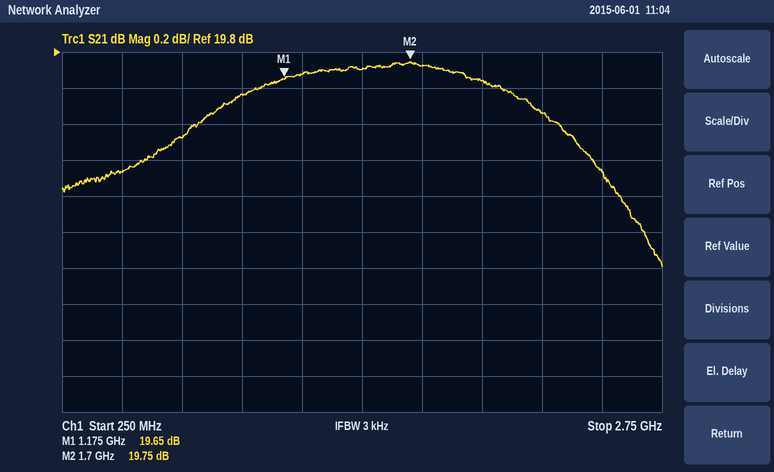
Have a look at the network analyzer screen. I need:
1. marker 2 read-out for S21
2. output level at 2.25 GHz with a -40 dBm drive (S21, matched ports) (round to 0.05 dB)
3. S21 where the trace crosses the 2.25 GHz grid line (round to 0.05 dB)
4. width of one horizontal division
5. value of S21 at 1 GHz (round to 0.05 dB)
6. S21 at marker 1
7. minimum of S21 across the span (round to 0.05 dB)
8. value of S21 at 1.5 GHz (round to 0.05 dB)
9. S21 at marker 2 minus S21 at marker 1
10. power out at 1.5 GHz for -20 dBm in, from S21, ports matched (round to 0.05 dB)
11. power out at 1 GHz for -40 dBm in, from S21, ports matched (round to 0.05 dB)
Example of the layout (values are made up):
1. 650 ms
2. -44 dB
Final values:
1. 19.75 dB
2. -20.55 dBm
3. 19.45 dB
4. 250 MHz
5. 19.55 dB
6. 19.65 dB
7. 18.60 dB
8. 19.70 dB
9. 0.10 dB
10. -0.30 dBm
11. -20.45 dBm
